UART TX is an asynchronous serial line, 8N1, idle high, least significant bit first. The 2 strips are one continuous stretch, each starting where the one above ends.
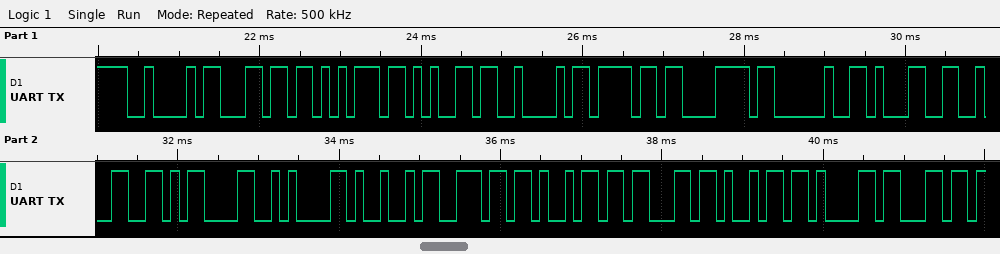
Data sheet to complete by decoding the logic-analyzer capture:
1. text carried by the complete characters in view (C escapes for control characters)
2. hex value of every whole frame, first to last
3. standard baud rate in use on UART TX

"BlueBox 12\r\nInicial"
42 6C 75 65 42 6F 78 20 31 32 0D 0A 49 6E 69 63 69 61 6C
9600 baud
